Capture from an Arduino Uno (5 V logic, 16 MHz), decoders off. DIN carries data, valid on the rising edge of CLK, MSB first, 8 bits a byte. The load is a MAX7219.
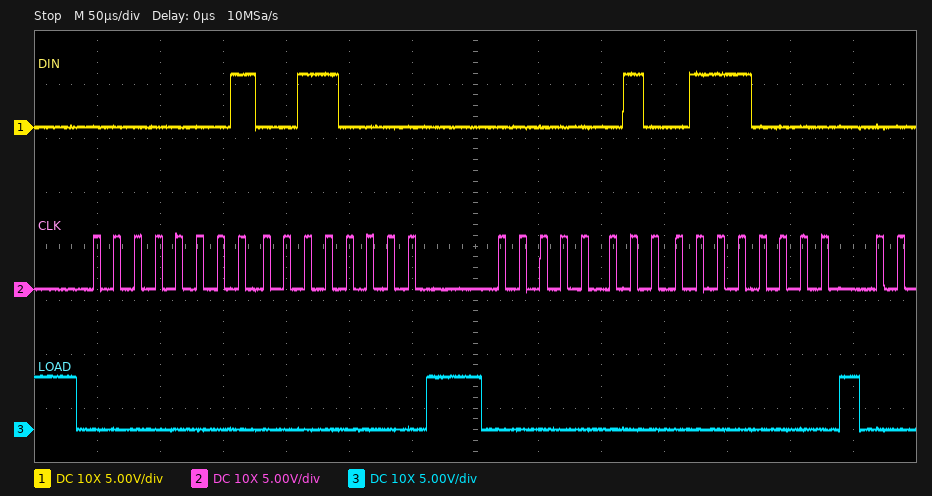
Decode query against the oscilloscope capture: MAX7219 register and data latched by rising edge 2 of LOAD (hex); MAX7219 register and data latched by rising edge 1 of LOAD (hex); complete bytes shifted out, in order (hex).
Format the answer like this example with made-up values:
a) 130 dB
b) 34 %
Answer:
a) register 0x2, data 0x70
b) register 0x1, data 0x30
c) 0x01 0x30 0x02 0x70
